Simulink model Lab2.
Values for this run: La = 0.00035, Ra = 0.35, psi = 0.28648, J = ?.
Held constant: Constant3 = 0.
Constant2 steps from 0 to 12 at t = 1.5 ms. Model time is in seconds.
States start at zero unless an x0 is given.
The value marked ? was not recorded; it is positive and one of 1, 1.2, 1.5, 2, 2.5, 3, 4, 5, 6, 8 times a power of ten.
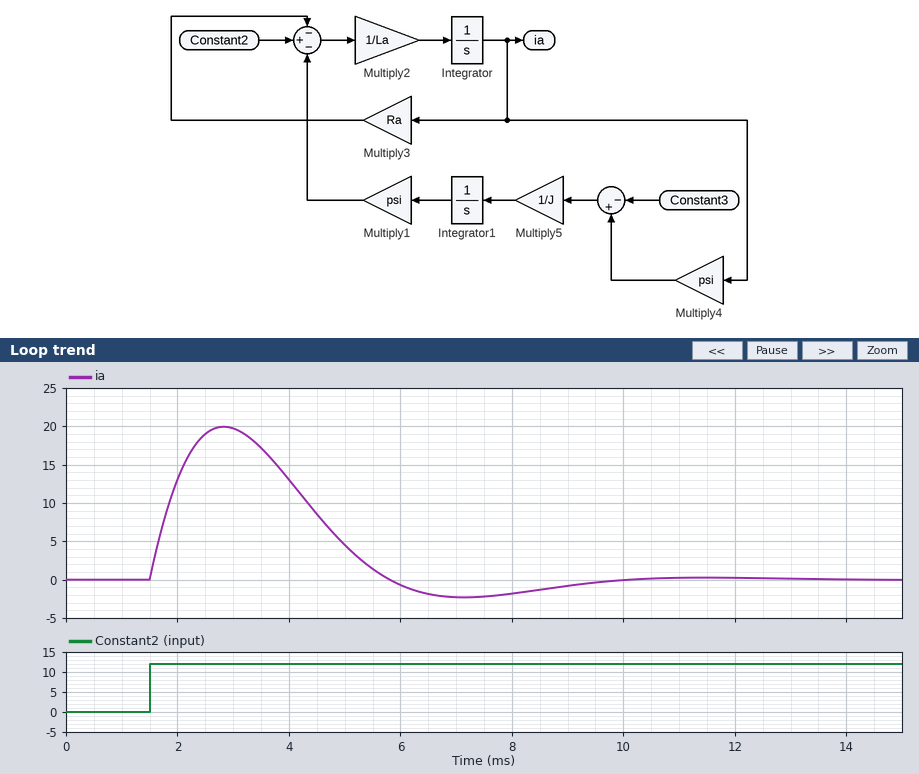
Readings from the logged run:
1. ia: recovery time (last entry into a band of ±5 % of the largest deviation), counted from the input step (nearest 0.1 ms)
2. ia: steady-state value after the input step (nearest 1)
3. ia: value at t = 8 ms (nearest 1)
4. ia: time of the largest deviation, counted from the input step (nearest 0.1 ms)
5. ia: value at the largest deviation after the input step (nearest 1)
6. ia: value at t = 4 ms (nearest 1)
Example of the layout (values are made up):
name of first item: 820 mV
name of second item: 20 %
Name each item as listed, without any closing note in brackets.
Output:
ia: recovery time (last entry into a band of ±5 % of the largest deviation), counted from the input step: 7.3 ms
ia: steady-state value after the input step: 0
ia: value at t = 8 ms: -2
ia: time of the largest deviation, counted from the input step: 1.3 ms
ia: value at the largest deviation after the input step: 20
ia: value at t = 4 ms: 13
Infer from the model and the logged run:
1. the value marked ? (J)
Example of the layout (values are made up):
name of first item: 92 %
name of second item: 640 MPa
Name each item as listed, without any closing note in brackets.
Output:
the value marked ?: 0.0003
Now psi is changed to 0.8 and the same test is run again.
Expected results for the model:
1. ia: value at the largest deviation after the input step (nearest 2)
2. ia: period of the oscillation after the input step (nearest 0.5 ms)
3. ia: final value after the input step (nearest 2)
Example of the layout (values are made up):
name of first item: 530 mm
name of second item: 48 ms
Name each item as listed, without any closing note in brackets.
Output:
ia: value at the largest deviation after the input step: 10
ia: period of the oscillation after the input step: 2.5 ms
ia: final value after the input step: 0
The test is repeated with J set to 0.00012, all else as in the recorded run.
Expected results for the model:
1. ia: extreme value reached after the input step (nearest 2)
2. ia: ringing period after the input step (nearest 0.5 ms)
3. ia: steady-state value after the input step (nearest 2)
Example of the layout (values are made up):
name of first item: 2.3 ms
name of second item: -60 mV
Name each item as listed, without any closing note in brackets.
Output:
ia: extreme value reached after the input step: 16
ia: ringing period after the input step: 5.0 ms
ia: steady-state value after the input step: 0
